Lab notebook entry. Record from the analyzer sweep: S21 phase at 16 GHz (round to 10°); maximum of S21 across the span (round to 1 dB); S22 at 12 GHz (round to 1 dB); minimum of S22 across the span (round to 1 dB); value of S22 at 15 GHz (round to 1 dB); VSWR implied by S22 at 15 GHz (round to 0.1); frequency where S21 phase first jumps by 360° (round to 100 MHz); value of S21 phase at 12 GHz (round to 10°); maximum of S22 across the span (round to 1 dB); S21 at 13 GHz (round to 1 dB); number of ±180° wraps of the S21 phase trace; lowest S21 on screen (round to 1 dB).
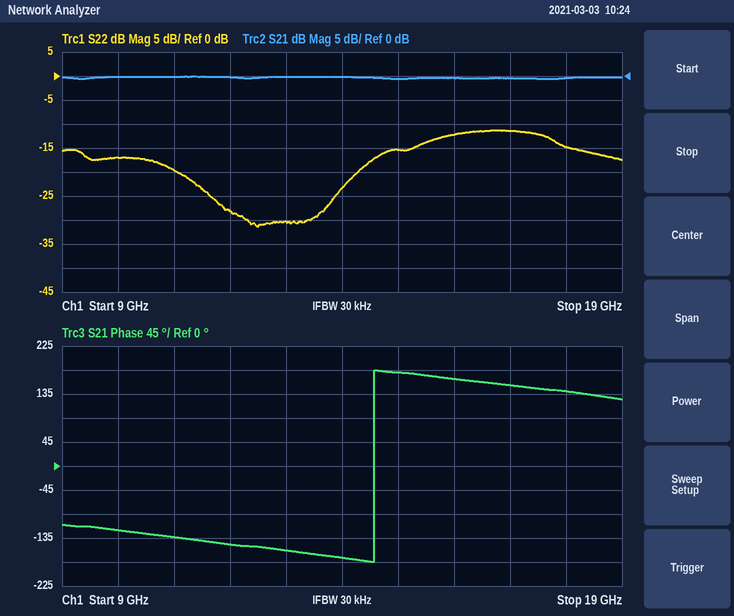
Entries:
160°
0 dB
-28 dB
-31 dB
-15 dB
1.4
14.6 GHz
-150°
-11 dB
0 dB
1
-1 dB
